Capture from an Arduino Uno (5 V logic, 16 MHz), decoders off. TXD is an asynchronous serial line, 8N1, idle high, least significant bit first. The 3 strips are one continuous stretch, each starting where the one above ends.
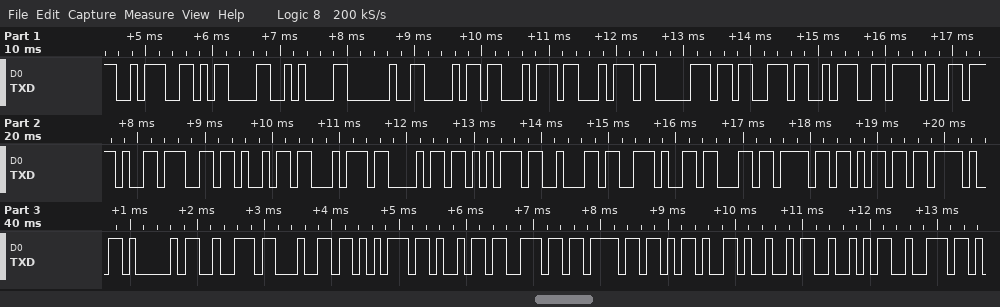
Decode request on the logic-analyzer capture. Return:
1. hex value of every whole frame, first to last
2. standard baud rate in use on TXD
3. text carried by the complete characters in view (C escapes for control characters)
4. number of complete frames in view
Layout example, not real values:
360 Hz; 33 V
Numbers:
3A 0D 0A 20 68 74 74 70 73 3A 2F 2F 67 69 74 68 75 62 2E 63 6F 6D 2F 41 72 64 75 69 6E 6F 2D 49 52 72; 9600 baud; ":\r\n https://github.com/Arduino-IRr"; 34
